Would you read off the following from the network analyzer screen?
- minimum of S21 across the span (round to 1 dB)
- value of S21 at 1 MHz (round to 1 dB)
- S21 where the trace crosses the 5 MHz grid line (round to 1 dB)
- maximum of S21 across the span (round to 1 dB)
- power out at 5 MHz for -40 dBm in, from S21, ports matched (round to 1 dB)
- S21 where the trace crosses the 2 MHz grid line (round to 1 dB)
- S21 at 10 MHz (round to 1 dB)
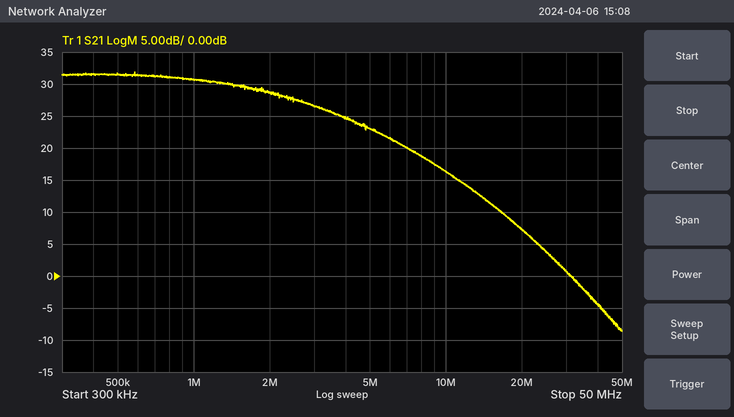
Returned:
-9 dB
31 dB
23 dB
32 dB
-17 dBm
29 dB
16 dB
